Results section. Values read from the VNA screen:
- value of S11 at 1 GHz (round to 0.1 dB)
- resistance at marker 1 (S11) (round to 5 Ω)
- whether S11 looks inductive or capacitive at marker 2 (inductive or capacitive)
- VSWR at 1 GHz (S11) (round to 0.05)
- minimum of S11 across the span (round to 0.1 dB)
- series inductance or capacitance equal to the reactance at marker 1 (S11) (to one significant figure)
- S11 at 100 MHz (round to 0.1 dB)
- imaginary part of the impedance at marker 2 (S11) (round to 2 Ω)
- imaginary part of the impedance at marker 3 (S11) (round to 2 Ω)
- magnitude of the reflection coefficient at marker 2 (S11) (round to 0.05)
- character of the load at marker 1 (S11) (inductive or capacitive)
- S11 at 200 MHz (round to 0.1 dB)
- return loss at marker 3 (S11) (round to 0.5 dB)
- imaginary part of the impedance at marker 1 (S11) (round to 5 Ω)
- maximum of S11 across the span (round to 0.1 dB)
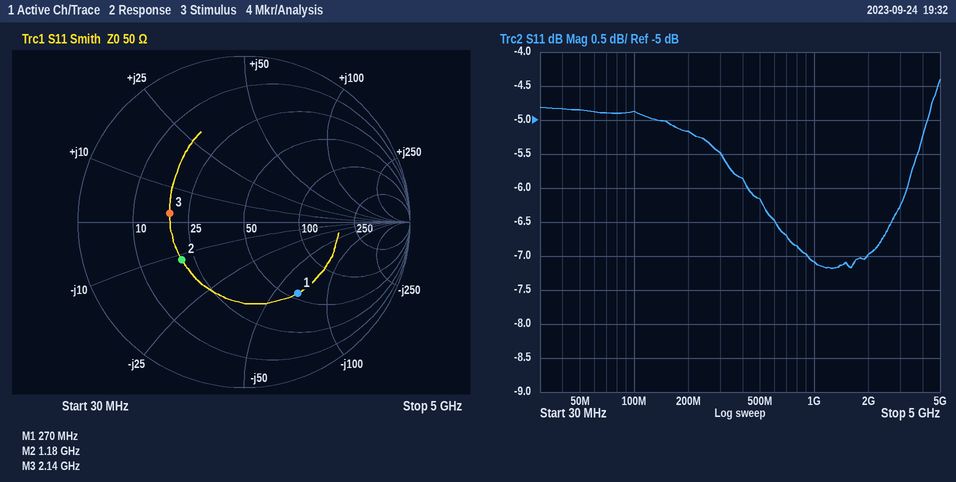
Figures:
-7.1 dB
55 Ω
capacitive
2.60
-7.2 dB
9 pF
-4.9 dB
-12 Ω
+2 Ω
0.45
capacitive
-5.2 dB
7.0 dB
-65 Ω
-4.4 dB
